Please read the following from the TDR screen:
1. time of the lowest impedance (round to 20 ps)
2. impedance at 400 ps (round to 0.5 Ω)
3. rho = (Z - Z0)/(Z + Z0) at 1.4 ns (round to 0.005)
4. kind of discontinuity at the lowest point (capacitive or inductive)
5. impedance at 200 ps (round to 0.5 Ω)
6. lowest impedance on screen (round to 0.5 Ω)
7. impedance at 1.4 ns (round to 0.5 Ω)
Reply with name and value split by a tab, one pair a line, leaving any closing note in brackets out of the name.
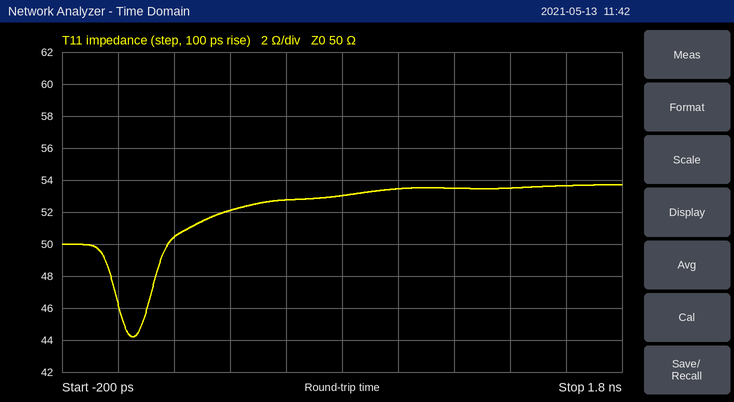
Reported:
time of the lowest impedance	60 ps
impedance at 400 ps	52.0 Ω
rho = (Z - Z0)/(Z + Z0) at 1.4 ns	+0.035
kind of discontinuity at the lowest point	capacitive
impedance at 200 ps	50.5 Ω
lowest impedance on screen	44.0 Ω
impedance at 1.4 ns	53.5 Ω
